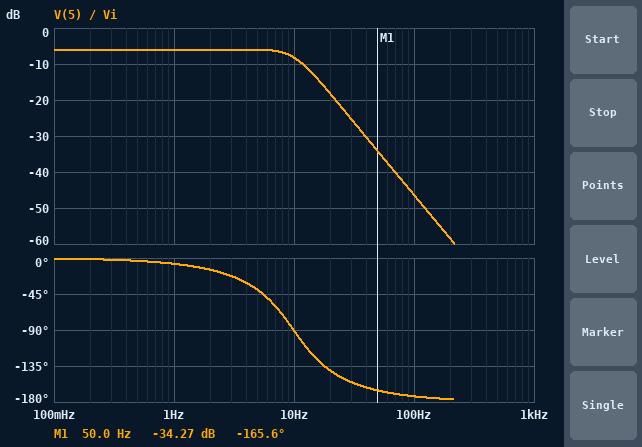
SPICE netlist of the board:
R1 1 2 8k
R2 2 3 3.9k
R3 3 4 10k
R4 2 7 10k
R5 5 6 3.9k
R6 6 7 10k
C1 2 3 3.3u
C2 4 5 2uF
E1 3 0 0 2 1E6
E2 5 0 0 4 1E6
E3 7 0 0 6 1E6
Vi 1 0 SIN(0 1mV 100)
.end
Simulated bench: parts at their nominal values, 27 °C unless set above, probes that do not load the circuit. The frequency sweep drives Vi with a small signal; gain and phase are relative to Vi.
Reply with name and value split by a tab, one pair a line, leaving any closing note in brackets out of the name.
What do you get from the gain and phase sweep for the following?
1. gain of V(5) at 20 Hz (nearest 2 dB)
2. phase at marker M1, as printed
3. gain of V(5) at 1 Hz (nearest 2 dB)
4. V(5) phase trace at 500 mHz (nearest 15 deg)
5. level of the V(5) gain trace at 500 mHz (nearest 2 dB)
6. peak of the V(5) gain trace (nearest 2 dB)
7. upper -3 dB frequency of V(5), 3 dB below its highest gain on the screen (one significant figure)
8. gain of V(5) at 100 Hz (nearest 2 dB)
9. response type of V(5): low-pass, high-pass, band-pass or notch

gain of V(5) at 20 Hz	-18 dB
phase at marker M1, as printed	-165.6 deg
gain of V(5) at 1 Hz	-6 dB
V(5) phase trace at 500 mHz	0 deg
level of the V(5) gain trace at 500 mHz	-6 dB
peak of the V(5) gain trace	-6 dB
upper -3 dB frequency of V(5), 3 dB below its highest gain on the screen	10 Hz
gain of V(5) at 100 Hz	-46 dB
response type of V(5): low-pass, high-pass, band-pass or notch	low-pass
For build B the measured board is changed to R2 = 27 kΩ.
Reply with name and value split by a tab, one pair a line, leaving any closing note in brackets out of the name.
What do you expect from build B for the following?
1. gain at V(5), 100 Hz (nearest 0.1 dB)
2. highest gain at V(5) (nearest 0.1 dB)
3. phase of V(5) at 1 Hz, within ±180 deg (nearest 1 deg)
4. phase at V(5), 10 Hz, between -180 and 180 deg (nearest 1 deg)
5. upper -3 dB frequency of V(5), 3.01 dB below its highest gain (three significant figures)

gain at V(5), 100 Hz	-46.3 dB
highest gain at V(5)	8.7 dB
phase of V(5) at 1 Hz, within ±180 deg	-1 deg
phase at V(5), 10 Hz, between -180 and 180 deg	-95 deg
upper -3 dB frequency of V(5), 3.01 dB below its highest gain	10.7 Hz
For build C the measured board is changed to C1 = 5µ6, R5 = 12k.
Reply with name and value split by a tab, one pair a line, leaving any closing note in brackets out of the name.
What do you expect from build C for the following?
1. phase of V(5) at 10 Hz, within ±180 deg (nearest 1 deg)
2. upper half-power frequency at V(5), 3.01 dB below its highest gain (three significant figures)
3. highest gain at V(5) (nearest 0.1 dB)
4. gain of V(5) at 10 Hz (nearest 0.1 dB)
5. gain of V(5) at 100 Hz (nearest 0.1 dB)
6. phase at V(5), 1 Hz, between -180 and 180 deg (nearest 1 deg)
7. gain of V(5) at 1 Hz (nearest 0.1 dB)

phase of V(5) at 10 Hz, within ±180 deg	-138 deg
upper half-power frequency at V(5), 3.01 dB below its highest gain	3.56 Hz
highest gain at V(5)	3.5 dB
gain of V(5) at 10 Hz	-11.7 dB
gain of V(5) at 100 Hz	-51.0 dB
phase at V(5), 1 Hz, between -180 and 180 deg	-22 deg
gain of V(5) at 1 Hz	3.3 dB
